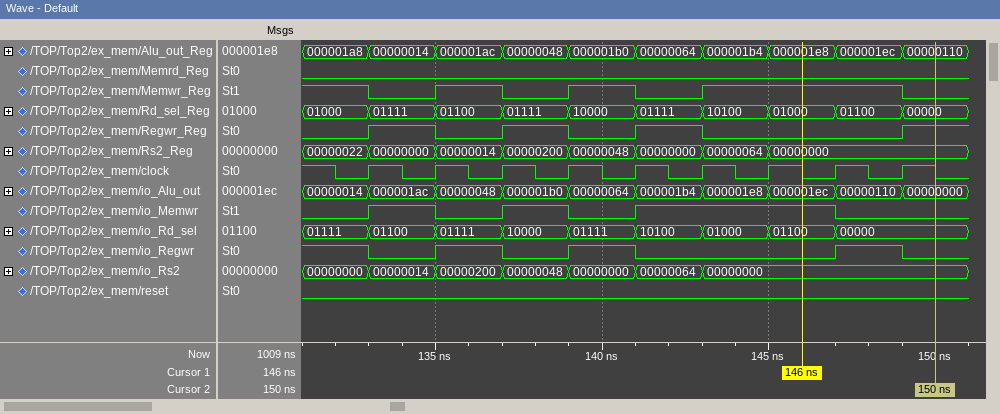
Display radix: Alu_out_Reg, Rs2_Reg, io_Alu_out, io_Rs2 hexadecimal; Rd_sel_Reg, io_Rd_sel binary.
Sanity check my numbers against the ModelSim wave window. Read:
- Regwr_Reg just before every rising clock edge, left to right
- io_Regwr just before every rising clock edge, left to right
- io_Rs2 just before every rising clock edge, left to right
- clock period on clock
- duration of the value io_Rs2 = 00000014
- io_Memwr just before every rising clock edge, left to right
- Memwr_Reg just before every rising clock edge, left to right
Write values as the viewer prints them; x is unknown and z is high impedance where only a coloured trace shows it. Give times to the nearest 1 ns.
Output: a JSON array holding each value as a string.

["0 1 0 1 0 1 0 0 0", "1 0 1 0 1 0 0 0 1", "00000000, 00000014, 00000200, 00000048, 00000000, 00000064, 00000000, 00000000, 00000000", "2 ns", "2 ns", "0 1 0 1 0 1 1 1 0", "1 0 1 0 1 0 1 1 1"]
